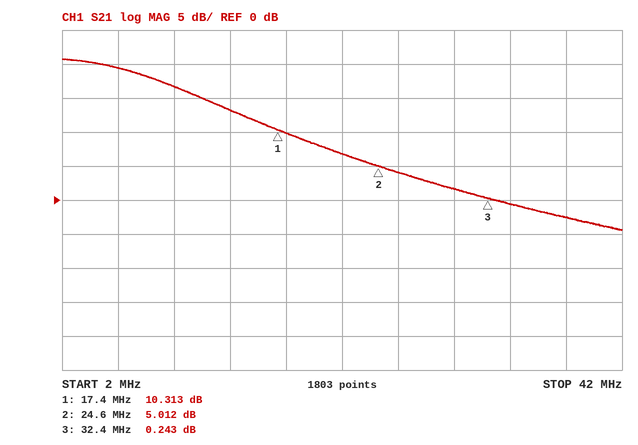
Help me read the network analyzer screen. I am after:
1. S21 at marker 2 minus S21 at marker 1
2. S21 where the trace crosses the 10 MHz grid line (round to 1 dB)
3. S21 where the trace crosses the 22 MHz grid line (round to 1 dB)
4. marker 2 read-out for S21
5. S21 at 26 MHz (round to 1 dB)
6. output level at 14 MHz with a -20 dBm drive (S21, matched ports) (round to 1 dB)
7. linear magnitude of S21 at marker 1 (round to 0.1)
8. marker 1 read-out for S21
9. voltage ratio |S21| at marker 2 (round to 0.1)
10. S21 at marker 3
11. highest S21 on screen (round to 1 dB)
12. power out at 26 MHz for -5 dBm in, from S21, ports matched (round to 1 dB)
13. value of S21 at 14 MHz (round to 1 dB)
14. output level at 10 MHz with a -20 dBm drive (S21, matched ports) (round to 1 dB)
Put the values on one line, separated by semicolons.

-5.301 dB; 17 dB; 7 dB; 5.012 dB; 4 dB; -7 dBm; 3.3; 10.313 dB; 1.8; 0.243 dB; 21 dB; -1 dBm; 13 dB; -3 dBm
